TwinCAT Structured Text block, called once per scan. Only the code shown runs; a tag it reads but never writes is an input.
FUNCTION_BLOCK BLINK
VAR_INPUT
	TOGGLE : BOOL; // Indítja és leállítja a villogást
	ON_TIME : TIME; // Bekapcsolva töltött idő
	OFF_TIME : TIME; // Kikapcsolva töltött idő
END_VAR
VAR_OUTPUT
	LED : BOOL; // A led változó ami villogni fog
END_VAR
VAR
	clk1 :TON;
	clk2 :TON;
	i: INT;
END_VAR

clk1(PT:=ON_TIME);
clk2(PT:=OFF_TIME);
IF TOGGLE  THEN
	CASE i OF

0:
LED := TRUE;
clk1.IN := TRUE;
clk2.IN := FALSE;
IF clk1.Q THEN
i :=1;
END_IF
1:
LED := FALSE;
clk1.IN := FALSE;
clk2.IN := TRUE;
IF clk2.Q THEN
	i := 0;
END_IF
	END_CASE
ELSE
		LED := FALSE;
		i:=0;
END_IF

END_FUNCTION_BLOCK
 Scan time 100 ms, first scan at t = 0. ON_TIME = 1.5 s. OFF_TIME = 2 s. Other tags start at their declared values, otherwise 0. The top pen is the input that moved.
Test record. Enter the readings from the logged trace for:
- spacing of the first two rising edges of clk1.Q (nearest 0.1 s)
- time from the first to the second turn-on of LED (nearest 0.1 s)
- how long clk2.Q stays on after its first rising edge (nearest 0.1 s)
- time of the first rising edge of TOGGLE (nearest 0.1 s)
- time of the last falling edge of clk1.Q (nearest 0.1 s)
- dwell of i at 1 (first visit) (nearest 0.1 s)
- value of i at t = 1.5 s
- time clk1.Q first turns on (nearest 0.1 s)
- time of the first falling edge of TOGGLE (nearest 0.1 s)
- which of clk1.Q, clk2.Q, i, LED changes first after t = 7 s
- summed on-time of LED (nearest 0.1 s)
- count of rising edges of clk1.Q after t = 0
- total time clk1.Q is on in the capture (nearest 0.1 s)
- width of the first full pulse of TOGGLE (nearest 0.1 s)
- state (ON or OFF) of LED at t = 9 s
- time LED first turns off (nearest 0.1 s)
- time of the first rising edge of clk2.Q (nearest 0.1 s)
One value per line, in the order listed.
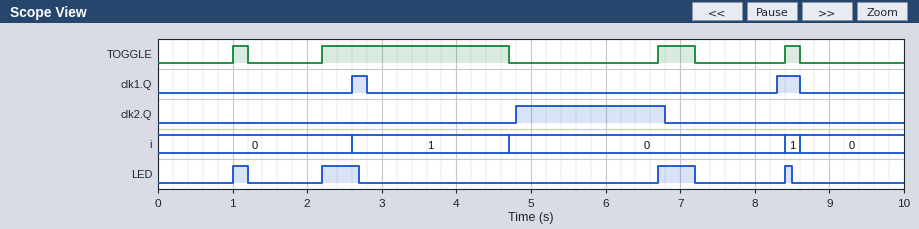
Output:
5.7 s
1.2 s
2.0 s
1.0 s
8.6 s
2.1 s
0
2.6 s
1.2 s
LED
1.3 s
2
0.5 s
0.2 s
OFF
1.2 s
4.8 s
